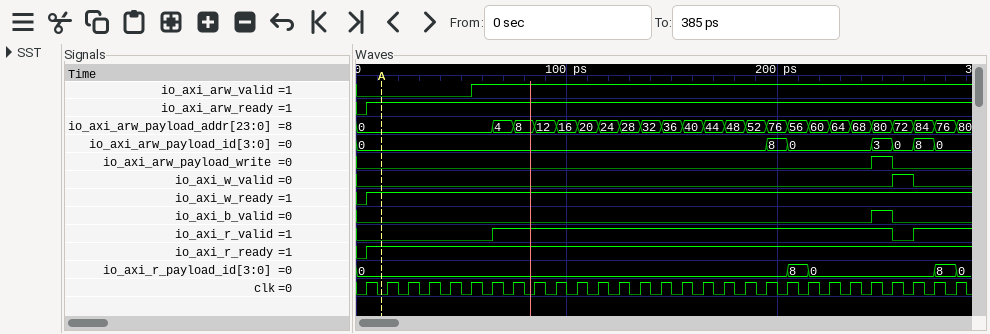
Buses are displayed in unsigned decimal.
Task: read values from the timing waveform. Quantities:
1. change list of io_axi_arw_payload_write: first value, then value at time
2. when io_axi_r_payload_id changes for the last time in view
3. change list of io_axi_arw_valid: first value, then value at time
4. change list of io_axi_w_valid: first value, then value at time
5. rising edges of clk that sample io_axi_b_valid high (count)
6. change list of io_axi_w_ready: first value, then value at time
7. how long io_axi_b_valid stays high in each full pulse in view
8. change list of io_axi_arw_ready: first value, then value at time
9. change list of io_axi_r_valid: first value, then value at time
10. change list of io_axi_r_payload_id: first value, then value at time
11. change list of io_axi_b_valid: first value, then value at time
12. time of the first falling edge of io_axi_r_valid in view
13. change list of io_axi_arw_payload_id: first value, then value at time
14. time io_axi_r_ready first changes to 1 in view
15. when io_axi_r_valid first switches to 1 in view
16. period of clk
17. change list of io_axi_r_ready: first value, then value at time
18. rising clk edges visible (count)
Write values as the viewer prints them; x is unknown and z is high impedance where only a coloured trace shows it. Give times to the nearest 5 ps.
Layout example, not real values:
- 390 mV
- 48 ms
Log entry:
- 0, 1 at 245 ps, 0 at 255 ps
- 285 ps
- 0, 1 at 55 ps
- 0, 1 at 255 ps, 0 at 265 ps
- 1
- 0, 1 at 5 ps
- 10 ps
- 0, 1 at 5 ps
- 0, 1 at 65 ps, 0 at 255 ps, 1 at 265 ps
- 0, 8 at 205 ps, 0 at 215 ps, 8 at 275 ps, 0 at 285 ps
- 0, 1 at 245 ps, 0 at 255 ps
- 255 ps
- 0, 8 at 195 ps, 0 at 205 ps, 3 at 245 ps, 0 at 255 ps, 8 at 265 ps, 0 at 275 ps
- 5 ps
- 65 ps
- 10 ps
- 0, 1 at 5 ps
- 29
